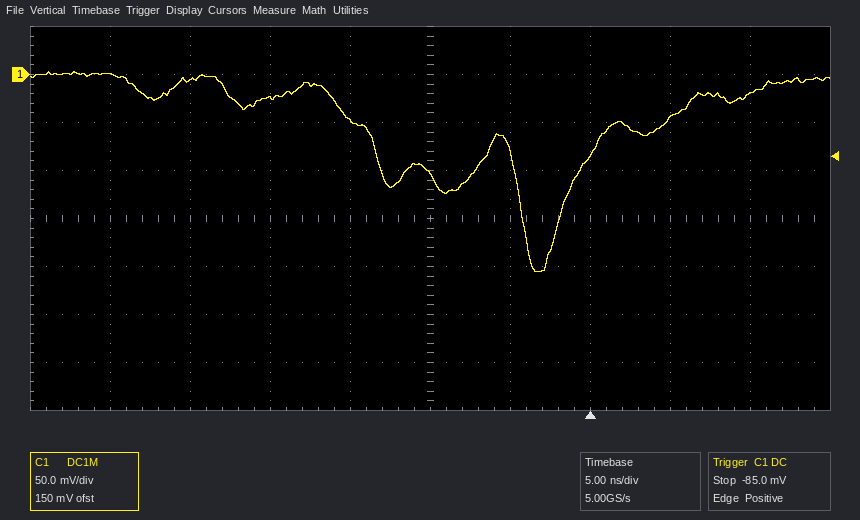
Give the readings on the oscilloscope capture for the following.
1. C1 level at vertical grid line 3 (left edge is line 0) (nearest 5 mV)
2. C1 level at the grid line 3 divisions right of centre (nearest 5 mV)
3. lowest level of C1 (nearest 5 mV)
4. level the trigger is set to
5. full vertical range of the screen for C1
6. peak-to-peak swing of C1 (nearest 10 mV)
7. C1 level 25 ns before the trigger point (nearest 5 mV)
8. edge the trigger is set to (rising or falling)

-25 mV
-45 mV
-205 mV
-85.0 mV
400 mV
210 mV
-5 mV
rising
